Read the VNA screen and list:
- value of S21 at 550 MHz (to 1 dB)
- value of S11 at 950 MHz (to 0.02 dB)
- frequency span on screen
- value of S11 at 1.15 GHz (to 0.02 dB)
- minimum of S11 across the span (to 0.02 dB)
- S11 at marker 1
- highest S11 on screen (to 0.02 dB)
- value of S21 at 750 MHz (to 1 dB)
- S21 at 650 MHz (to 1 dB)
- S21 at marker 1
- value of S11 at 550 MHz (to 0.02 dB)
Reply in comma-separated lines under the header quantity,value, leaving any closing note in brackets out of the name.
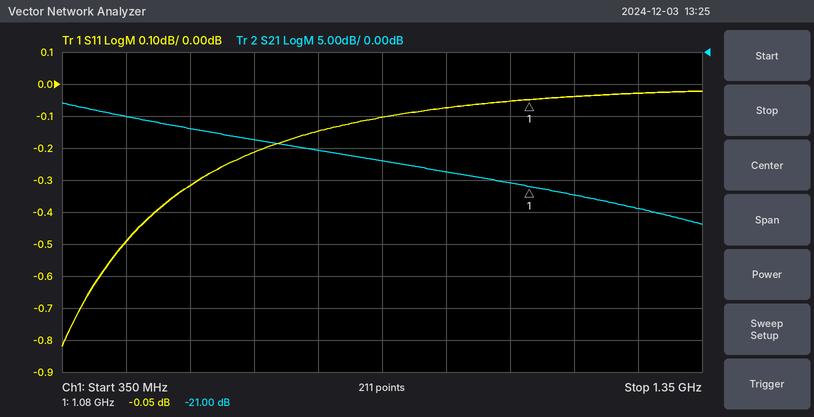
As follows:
quantity,value
value of S21 at 550 MHz,-12 dB
value of S11 at 950 MHz,-0.08 dB
frequency span on screen,1 GHz
value of S11 at 1.15 GHz,-0.04 dB
minimum of S11 across the span,-0.82 dB
S11 at marker 1,-0.05 dB
highest S11 on screen,-0.02 dB
value of S21 at 750 MHz,-15 dB
S21 at 650 MHz,-14 dB
S21 at marker 1,-21.00 dB
value of S11 at 550 MHz,-0.32 dB
